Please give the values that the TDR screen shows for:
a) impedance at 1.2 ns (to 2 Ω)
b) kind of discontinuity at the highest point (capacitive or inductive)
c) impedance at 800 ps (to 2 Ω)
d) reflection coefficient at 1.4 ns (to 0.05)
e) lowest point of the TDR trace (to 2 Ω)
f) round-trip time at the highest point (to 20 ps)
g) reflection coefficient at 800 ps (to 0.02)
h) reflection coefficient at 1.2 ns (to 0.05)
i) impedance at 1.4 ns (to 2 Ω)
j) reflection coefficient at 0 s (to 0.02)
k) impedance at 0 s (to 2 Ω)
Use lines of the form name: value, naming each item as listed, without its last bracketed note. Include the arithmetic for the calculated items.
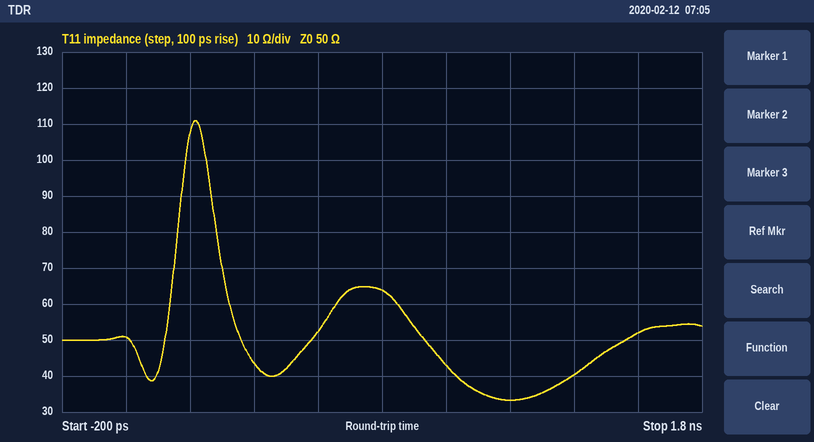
impedance at 1.2 ns: 34 Ω
kind of discontinuity at the highest point: inductive
impedance at 800 ps: 64 Ω
reflection coefficient at 1.4 ns: (40 − 50)/(40 + 50) ≈ -0.111, so -0.10 to the nearest 0.05
lowest point of the TDR trace: 34 Ω
round-trip time at the highest point: 220 ps
reflection coefficient at 800 ps: (64 − 50)/(64 + 50) ≈ +0.12
reflection coefficient at 1.2 ns: (34 − 50)/(34 + 50) ≈ -0.190, so -0.20 to the nearest 0.05
impedance at 1.4 ns: 40 Ω
reflection coefficient at 0 s: (50 − 50)/(50 + 50) ≈ 0.00
impedance at 0 s: 50 Ω
